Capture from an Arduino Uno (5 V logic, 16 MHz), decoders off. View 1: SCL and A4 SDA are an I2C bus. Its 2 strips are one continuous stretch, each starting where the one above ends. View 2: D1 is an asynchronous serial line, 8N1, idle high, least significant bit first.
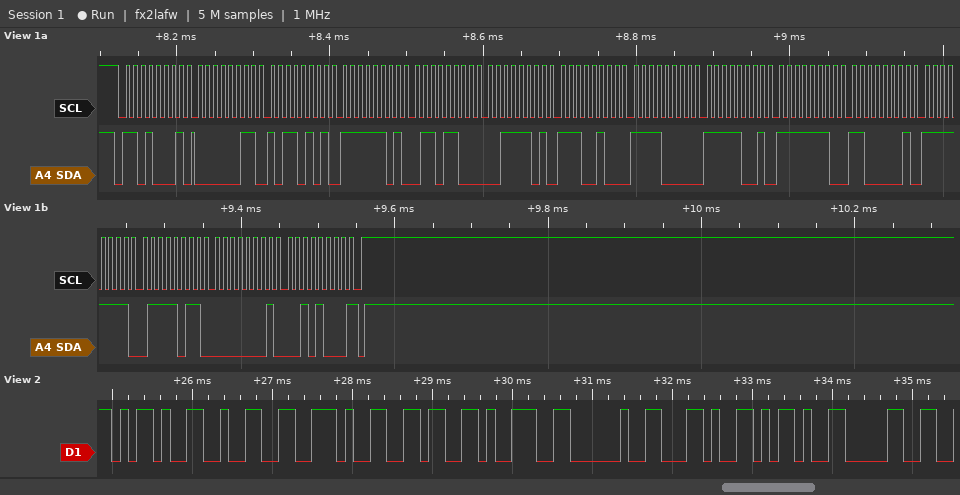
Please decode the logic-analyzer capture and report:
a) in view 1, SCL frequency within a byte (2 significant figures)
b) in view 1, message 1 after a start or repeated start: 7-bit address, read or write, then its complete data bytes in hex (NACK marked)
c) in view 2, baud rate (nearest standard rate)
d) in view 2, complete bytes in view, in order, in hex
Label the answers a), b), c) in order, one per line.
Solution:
a) 100 kHz
b) 0x68 read: 03 B5 FD 6C 3D E4 F0 F9 FE C1 FF 7B 01 28 NACK
c) 9600 baud
d) 2D 32 2E 36 39 20 2C 2D 30
